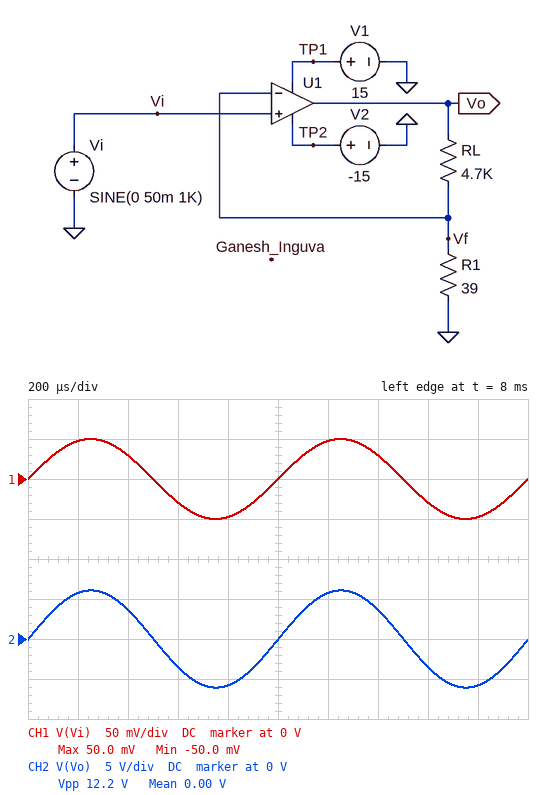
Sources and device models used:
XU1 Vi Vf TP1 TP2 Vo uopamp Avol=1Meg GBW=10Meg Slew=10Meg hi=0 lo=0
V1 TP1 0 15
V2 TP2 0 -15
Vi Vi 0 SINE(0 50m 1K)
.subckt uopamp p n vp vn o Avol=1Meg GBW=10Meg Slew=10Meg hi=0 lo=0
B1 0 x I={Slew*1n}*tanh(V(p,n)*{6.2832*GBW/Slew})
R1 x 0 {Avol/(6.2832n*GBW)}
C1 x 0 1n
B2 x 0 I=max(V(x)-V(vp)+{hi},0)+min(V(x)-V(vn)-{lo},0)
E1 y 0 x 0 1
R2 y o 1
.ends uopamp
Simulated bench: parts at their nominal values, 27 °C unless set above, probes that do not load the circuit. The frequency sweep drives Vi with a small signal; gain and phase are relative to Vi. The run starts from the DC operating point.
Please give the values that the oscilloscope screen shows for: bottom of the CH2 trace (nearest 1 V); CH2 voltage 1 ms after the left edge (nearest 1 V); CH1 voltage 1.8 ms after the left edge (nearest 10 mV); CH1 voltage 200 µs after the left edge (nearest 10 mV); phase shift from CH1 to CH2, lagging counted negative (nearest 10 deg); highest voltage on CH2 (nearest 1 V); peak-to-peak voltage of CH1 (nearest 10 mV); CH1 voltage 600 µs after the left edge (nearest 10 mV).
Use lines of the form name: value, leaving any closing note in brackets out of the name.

bottom of the CH2 trace: -6 V
CH2 voltage 1 ms after the left edge: 0 V
CH1 voltage 1.8 ms after the left edge: -50 mV
CH1 voltage 200 µs after the left edge: 50 mV
phase shift from CH1 to CH2, lagging counted negative: 0 deg
highest voltage on CH2: 6 V
peak-to-peak voltage of CH1: 100 mV
CH1 voltage 600 µs after the left edge: -30 mV
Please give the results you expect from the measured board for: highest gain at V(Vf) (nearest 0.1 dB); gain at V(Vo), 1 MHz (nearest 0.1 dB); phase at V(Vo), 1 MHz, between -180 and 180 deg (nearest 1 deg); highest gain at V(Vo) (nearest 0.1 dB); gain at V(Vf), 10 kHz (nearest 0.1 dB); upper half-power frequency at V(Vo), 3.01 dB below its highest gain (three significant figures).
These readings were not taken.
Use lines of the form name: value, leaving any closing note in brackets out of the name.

highest gain at V(Vf): 0 dB
gain at V(Vo), 1 MHz: 20.0 dB
phase at V(Vo), 1 MHz, between -180 and 180 deg: -85 deg
highest gain at V(Vo): 41.7 dB
gain at V(Vf), 10 kHz: -0.1 dB
upper half-power frequency at V(Vo), 3.01 dB below its highest gain: 82.3 kHz
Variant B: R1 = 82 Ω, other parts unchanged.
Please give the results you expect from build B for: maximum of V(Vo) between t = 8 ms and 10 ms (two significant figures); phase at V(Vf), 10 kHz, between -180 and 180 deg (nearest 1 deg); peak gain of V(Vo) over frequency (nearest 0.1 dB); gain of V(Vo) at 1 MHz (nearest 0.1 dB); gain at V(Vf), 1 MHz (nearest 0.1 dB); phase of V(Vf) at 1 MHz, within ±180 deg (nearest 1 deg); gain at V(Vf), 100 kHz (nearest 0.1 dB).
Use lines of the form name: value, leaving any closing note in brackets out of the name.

maximum of V(Vo) between t = 8 ms and 10 ms: 2.9 V
phase at V(Vf), 10 kHz, between -180 and 180 deg: -3 deg
peak gain of V(Vo) over frequency: 35.3 dB
gain of V(Vo) at 1 MHz: 19.9 dB
gain at V(Vf), 1 MHz: -15.4 dB
phase of V(Vf) at 1 MHz, within ±180 deg: -80 deg
gain at V(Vf), 100 kHz: -1.3 dB
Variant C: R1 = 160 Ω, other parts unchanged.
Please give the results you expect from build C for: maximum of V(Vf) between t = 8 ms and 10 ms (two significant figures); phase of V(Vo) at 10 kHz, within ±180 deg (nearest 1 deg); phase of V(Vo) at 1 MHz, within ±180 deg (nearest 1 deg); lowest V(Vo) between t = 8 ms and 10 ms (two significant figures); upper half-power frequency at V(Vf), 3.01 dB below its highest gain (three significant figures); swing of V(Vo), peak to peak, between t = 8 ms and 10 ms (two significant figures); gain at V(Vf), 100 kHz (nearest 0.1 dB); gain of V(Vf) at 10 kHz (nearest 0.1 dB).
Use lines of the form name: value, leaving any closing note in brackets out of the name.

maximum of V(Vf) between t = 8 ms and 10 ms: 50 mV
phase of V(Vo) at 10 kHz, within ±180 deg: -2 deg
phase of V(Vo) at 1 MHz, within ±180 deg: -72 deg
lowest V(Vo) between t = 8 ms and 10 ms: -1.5 V
upper half-power frequency at V(Vf), 3.01 dB below its highest gain: 329 kHz
swing of V(Vo), peak to peak, between t = 8 ms and 10 ms: 3.0 V
gain at V(Vf), 100 kHz: -0.4 dB
gain of V(Vf) at 10 kHz: 0 dB
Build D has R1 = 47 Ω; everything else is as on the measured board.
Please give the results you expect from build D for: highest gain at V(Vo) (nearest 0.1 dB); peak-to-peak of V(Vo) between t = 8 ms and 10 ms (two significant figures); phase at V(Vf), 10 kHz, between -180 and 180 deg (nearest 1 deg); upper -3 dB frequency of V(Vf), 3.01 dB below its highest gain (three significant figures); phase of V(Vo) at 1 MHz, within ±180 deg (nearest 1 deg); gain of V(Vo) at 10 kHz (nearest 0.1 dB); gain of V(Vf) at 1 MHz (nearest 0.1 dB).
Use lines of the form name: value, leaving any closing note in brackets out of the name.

highest gain at V(Vo): 40.1 dB
peak-to-peak of V(Vo) between t = 8 ms and 10 ms: 10 V
phase at V(Vf), 10 kHz, between -180 and 180 deg: -6 deg
upper -3 dB frequency of V(Vf), 3.01 dB below its highest gain: 99.0 kHz
phase of V(Vo) at 1 MHz, within ±180 deg: -84 deg
gain of V(Vo) at 10 kHz: 40.0 dB
gain of V(Vf) at 1 MHz: -20.1 dB
